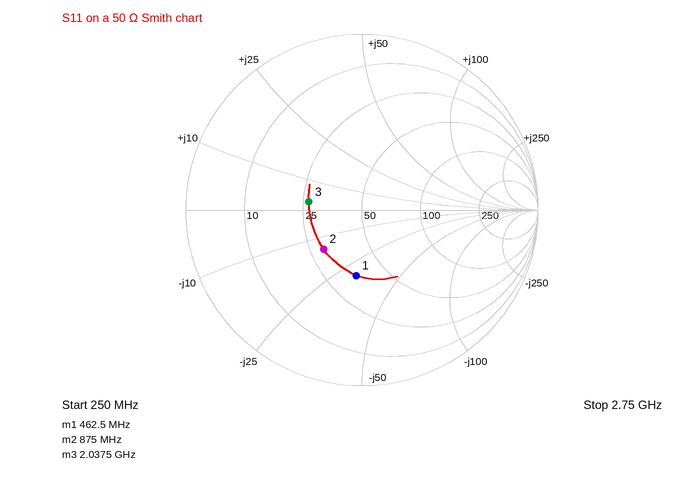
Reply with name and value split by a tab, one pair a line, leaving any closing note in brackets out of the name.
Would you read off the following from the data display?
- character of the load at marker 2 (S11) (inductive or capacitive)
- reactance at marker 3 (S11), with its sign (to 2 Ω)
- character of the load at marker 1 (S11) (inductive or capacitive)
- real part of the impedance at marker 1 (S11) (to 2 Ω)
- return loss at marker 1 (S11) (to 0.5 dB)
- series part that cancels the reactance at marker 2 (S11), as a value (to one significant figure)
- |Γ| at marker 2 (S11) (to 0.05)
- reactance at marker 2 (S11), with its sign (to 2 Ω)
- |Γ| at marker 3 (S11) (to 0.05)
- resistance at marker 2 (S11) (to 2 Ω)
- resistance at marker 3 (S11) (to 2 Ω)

character of the load at marker 2 (S11)	capacitive
reactance at marker 3 (S11), with its sign	+2 Ω
character of the load at marker 1 (S11)	capacitive
real part of the impedance at marker 1 (S11)	36 Ω
return loss at marker 1 (S11)	8.5 dB
series part that cancels the reactance at marker 2 (S11), as a value	3 nH
|Γ| at marker 2 (S11)	0.30
reactance at marker 2 (S11), with its sign	-14 Ω
|Γ| at marker 3 (S11)	0.30
resistance at marker 2 (S11)	30 Ω
resistance at marker 3 (S11)	26 Ω
